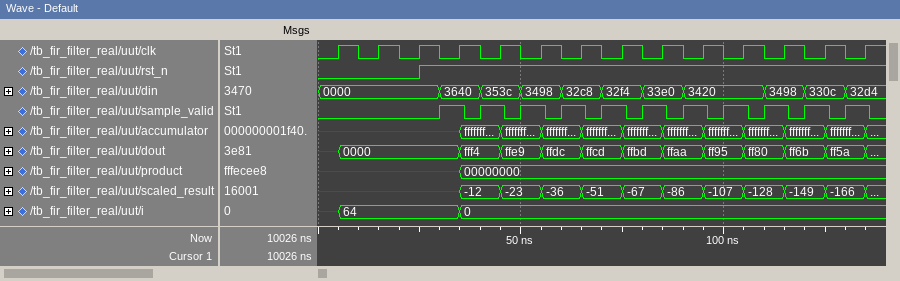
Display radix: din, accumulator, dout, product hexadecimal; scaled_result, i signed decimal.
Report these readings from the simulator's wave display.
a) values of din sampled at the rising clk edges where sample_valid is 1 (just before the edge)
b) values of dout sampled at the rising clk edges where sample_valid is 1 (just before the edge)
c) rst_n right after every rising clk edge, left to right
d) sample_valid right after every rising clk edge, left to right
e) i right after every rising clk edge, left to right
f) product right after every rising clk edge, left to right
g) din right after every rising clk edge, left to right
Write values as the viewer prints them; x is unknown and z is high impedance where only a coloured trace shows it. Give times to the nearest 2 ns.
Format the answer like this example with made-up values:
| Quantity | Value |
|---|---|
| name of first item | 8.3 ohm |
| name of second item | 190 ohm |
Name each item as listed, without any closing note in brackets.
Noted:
| Quantity | Value |
|---|---|
| values of din sampled at the rising clk edges where sample_valid is 1 | 3640, 353c, 3498, 32c8, 32f4, 33e0, 3420, 3420, 3498, 330c, 32d4 |
| values of dout sampled at the rising clk edges where sample_valid is 1 | 0000, fff4, ffe9, ffdc, ffcd, ffbd, ffaa, ff95, ff80, ff6b, ff5a |
| rst_n right after every rising clk edge, left to right | 0 0 1 1 1 1 1 1 1 1 1 1 1 1 |
| sample_valid right after every rising clk edge, left to right | 0 0 0 1 1 1 1 1 1 1 1 1 1 1 |
| i right after every rising clk edge, left to right | 64, 64, 64, 0, 0, 0, 0, 0, 0, 0, 0, 0, 0, 0 |
| product right after every rising clk edge, left to right | x, x, x, 00000000, 00000000, 00000000, 00000000, 00000000, 00000000, 00000000, 00000000, 00000000, 00000000, 00000000 |
| din right after every rising clk edge, left to right | 0000, 0000, 0000, 3640, 353c, 3498, 32c8, 32f4, 33e0, 3420, 3420, 3498, 330c, 32d4 |
